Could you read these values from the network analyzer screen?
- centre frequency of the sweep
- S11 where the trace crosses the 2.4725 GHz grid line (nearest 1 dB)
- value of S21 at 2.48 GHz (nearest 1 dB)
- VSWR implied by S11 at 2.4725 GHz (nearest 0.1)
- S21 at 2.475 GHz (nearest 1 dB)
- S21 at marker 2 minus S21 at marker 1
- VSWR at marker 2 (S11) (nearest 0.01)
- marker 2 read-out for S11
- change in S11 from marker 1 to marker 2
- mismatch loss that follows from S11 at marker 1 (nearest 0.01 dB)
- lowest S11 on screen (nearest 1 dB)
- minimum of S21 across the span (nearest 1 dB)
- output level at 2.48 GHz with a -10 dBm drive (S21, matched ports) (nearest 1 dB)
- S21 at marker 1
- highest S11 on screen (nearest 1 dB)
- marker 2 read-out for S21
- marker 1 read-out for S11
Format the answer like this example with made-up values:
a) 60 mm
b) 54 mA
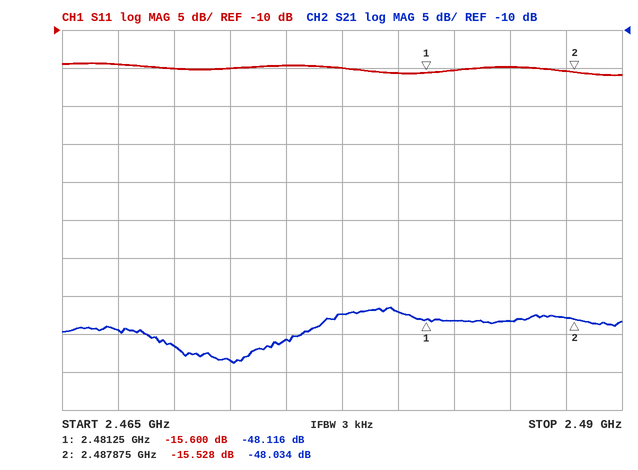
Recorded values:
a) 2.4775 GHz
b) -15 dB
c) -47 dB
d) 1.4
e) -51 dB
f) 0.082 dB
g) 1.40
h) -15.528 dB
i) 0.072 dB
j) 0.12 dB
k) -16 dB
l) -54 dB
m) -57 dBm
n) -48.116 dB
o) -14 dB
p) -48.034 dB
q) -15.600 dB
